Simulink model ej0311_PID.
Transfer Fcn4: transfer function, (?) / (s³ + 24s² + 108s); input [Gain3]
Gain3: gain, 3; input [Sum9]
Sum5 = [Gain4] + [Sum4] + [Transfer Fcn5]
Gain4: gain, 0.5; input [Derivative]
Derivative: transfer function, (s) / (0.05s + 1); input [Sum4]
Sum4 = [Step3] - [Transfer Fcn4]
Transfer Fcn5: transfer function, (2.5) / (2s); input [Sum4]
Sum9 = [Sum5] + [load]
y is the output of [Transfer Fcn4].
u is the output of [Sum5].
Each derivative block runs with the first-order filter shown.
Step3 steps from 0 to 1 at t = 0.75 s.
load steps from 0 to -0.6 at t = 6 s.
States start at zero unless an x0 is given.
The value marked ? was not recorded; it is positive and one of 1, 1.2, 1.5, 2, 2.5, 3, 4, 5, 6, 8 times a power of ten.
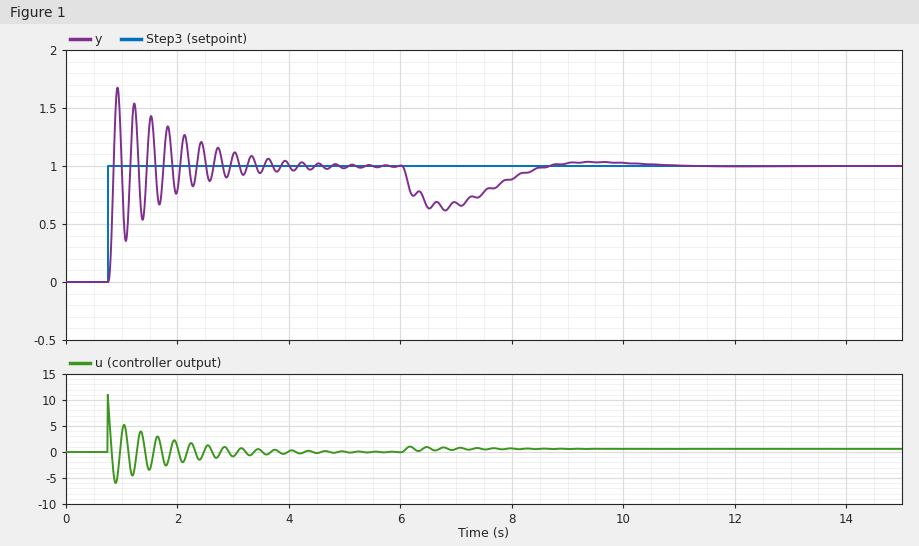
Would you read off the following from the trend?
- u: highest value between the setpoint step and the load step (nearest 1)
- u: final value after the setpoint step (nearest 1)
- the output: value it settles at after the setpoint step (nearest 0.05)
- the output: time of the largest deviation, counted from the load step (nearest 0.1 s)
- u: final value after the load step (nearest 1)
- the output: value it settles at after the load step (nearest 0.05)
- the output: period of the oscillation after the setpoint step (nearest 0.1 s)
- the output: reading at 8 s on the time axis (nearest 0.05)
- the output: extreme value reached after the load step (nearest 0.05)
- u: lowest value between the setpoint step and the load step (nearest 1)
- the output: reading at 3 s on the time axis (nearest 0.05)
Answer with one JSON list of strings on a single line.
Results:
["11", "0", "1.00", "0.8 s", "1", "1.00", "0.3 s", "0.90", "0.60", "-6", "1.10"]
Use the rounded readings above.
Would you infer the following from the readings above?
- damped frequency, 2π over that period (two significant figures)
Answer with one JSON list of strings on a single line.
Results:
["21 rad/s"]
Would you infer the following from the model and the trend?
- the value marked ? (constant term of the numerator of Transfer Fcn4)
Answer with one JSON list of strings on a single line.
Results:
["500"]
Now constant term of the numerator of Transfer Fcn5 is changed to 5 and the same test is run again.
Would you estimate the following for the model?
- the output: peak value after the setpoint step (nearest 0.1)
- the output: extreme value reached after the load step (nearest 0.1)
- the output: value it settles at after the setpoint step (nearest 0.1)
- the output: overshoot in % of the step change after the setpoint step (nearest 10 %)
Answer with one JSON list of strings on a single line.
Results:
["1.7", "0.7", "1.0", "70 %"]
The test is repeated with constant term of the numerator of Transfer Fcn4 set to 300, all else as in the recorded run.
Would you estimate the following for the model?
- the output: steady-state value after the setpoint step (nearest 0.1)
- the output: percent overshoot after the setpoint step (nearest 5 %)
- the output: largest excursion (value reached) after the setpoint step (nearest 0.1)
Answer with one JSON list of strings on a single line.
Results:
["1.0", "40 %", "1.4"]
